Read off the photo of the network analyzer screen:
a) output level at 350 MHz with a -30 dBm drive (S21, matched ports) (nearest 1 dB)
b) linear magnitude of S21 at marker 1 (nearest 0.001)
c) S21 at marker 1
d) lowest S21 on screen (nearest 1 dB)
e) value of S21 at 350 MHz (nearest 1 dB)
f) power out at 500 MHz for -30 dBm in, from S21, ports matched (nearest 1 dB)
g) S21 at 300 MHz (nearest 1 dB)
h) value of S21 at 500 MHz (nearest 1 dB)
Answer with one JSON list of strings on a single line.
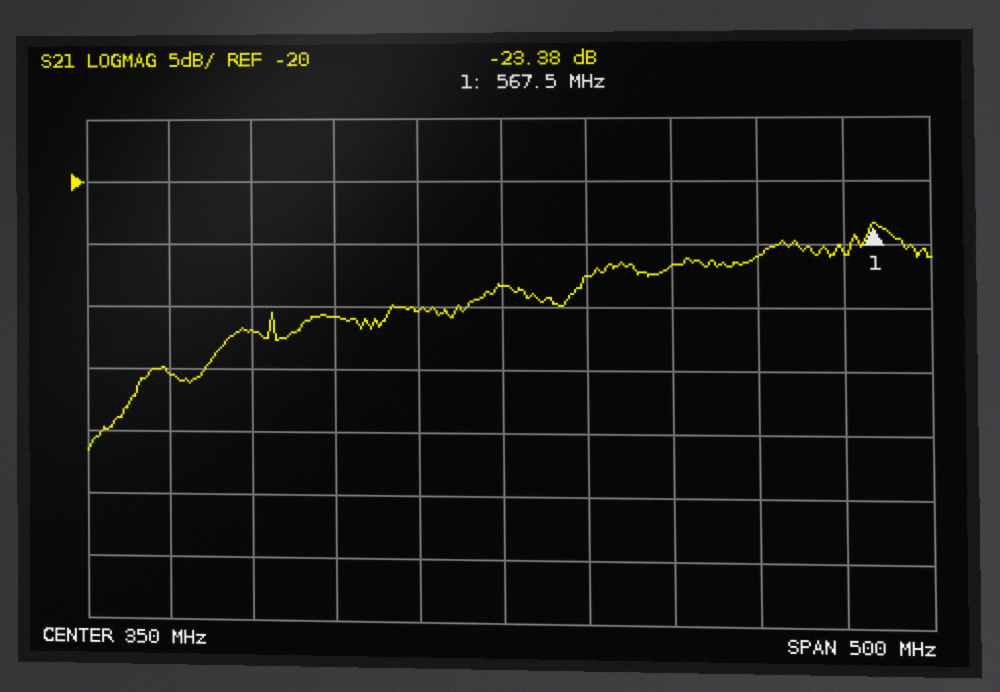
["-58 dBm", "0.068", "-23.38 dB", "-42 dB", "-28 dB", "-56 dBm", "-30 dB", "-26 dB"]
